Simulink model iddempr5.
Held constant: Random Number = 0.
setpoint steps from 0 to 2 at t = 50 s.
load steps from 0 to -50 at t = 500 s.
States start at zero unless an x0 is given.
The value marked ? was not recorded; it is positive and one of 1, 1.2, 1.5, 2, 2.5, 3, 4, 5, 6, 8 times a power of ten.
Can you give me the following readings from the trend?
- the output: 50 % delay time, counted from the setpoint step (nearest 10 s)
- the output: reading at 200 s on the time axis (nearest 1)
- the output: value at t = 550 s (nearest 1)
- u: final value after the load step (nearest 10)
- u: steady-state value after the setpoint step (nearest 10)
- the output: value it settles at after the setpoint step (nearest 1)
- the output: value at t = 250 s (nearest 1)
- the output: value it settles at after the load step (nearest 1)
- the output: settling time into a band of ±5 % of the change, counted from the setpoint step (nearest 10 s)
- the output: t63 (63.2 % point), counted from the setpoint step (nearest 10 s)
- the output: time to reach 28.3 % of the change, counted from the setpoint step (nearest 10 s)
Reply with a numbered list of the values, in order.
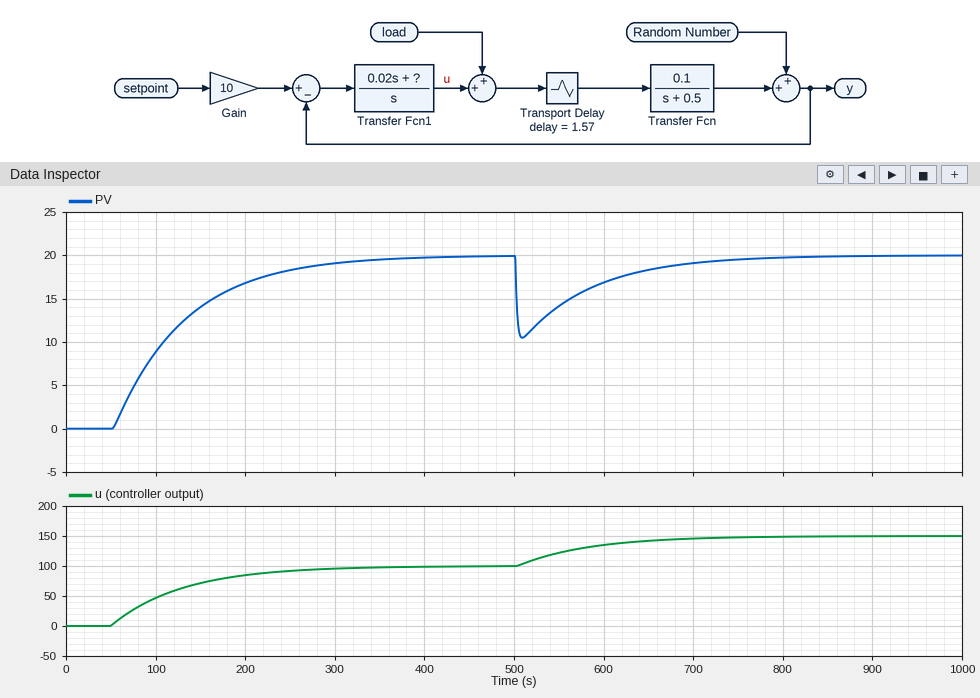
1. 60 s
2. 17
3. 14
4. 150
5. 100
6. 20
7. 18
8. 20
9. 240 s
10. 80 s
11. 30 s
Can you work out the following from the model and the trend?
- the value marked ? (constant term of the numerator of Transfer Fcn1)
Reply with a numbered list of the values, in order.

1. 0.06
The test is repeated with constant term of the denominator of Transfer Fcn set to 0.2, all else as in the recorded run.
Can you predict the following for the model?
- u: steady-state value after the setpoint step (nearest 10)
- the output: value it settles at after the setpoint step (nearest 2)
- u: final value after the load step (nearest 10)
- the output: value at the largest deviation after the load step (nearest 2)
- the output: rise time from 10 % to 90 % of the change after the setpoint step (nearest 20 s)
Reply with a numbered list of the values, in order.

1. 40
2. 20
3. 90
4. 0
5. 60 s
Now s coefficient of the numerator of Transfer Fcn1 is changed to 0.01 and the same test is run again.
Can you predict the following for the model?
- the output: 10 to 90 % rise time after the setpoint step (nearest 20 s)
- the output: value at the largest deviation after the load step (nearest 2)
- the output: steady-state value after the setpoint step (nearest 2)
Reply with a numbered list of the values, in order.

1. 180 s
2. 10
3. 20
